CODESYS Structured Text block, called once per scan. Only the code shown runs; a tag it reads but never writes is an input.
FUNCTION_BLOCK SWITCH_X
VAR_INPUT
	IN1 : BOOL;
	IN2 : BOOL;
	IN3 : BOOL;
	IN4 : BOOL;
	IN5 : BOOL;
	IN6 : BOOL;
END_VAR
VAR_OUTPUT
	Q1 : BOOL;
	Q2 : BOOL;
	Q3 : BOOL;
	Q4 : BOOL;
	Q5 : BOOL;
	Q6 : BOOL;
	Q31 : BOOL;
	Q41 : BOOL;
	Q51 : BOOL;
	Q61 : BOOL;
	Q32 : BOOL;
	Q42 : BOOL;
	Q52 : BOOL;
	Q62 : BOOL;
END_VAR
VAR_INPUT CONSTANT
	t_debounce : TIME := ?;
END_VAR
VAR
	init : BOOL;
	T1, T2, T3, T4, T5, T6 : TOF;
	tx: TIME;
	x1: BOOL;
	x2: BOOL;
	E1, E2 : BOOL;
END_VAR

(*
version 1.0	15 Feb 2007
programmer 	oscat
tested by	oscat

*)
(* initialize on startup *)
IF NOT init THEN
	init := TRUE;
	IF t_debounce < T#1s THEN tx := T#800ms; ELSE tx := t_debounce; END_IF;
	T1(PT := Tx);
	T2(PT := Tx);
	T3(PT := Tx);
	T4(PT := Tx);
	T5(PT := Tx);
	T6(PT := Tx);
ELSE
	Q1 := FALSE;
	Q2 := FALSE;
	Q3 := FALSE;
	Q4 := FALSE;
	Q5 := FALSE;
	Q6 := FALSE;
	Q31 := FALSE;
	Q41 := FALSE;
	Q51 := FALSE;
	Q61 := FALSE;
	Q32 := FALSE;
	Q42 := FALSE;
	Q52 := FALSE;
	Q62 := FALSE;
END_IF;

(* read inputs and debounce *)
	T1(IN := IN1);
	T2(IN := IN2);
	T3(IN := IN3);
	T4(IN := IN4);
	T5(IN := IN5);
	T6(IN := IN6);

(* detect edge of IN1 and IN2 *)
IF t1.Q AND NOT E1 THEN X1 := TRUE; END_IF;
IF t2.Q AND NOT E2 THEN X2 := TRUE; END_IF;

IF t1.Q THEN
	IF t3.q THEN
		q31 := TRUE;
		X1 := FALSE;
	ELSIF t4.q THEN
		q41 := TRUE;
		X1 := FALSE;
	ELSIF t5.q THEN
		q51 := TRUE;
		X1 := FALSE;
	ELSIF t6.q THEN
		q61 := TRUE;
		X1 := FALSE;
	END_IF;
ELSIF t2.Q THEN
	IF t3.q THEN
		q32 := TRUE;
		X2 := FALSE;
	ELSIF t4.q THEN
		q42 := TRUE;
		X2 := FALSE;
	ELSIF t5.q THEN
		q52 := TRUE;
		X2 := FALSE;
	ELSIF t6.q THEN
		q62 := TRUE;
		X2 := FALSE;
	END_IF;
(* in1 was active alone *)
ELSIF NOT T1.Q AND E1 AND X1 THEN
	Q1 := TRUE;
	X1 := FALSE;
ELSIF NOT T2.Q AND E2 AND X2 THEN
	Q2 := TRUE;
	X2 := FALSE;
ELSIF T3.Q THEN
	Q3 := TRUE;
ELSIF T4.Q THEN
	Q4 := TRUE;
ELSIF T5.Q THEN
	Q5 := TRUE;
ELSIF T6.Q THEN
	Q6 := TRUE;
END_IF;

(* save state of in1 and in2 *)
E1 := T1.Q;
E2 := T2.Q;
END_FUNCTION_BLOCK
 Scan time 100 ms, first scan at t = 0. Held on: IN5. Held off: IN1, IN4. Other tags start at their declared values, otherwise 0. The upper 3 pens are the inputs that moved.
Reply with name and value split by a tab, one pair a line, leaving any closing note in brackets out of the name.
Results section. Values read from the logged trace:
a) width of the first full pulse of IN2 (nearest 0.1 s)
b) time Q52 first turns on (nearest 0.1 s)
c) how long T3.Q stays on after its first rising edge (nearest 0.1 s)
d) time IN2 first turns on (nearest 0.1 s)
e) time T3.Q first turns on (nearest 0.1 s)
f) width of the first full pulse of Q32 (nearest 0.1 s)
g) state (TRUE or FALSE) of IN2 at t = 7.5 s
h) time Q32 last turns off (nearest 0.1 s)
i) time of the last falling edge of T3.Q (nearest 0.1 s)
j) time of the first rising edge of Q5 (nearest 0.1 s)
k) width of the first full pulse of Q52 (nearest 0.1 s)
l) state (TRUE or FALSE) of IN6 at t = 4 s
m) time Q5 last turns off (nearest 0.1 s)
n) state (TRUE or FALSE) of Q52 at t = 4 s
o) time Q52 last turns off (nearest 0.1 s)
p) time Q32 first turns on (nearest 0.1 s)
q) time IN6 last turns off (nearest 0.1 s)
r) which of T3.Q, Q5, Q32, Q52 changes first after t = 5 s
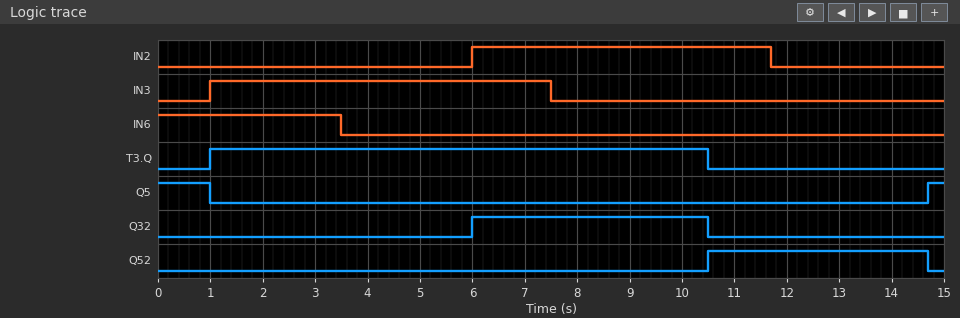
width of the first full pulse of IN2	5.7 s
time Q52 first turns on	10.5 s
how long T3.Q stays on after its first rising edge	9.5 s
time IN2 first turns on	6.0 s
time T3.Q first turns on	1.0 s
width of the first full pulse of Q32	4.5 s
state (TRUE or FALSE) of IN2 at t = 7.5 s	TRUE
time Q32 last turns off	10.5 s
time of the last falling edge of T3.Q	10.5 s
time of the first rising edge of Q5	14.7 s
width of the first full pulse of Q52	4.2 s
state (TRUE or FALSE) of IN6 at t = 4 s	FALSE
time Q5 last turns off	1.0 s
state (TRUE or FALSE) of Q52 at t = 4 s	FALSE
time Q52 last turns off	14.7 s
time Q32 first turns on	6.0 s
time IN6 last turns off	3.5 s
which of T3.Q, Q5, Q32, Q52 changes first after t = 5 s	Q32
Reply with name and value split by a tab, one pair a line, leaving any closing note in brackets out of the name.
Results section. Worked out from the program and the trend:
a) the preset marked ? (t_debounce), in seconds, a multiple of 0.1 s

the preset marked ? (t_debounce), in seconds, a multiple of 0.1 s	3.0 s
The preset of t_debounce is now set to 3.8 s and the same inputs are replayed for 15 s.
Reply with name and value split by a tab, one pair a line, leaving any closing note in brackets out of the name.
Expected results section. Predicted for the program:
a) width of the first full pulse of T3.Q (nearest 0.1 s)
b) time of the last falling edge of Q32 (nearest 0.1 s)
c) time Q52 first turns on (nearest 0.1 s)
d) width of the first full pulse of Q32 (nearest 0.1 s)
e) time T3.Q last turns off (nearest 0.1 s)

width of the first full pulse of T3.Q	10.3 s
time of the last falling edge of Q32	11.3 s
time Q52 first turns on	11.3 s
width of the first full pulse of Q32	5.3 s
time T3.Q last turns off	11.3 s
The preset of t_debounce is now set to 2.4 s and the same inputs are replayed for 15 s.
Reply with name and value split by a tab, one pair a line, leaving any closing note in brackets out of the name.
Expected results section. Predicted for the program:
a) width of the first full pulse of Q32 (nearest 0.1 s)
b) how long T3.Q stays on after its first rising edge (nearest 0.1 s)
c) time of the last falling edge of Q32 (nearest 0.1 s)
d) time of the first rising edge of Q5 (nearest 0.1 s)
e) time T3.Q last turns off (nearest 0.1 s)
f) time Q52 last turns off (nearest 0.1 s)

width of the first full pulse of Q32	3.9 s
how long T3.Q stays on after its first rising edge	8.9 s
time of the last falling edge of Q32	9.9 s
time of the first rising edge of Q5	14.1 s
time T3.Q last turns off	9.9 s
time Q52 last turns off	14.1 s
